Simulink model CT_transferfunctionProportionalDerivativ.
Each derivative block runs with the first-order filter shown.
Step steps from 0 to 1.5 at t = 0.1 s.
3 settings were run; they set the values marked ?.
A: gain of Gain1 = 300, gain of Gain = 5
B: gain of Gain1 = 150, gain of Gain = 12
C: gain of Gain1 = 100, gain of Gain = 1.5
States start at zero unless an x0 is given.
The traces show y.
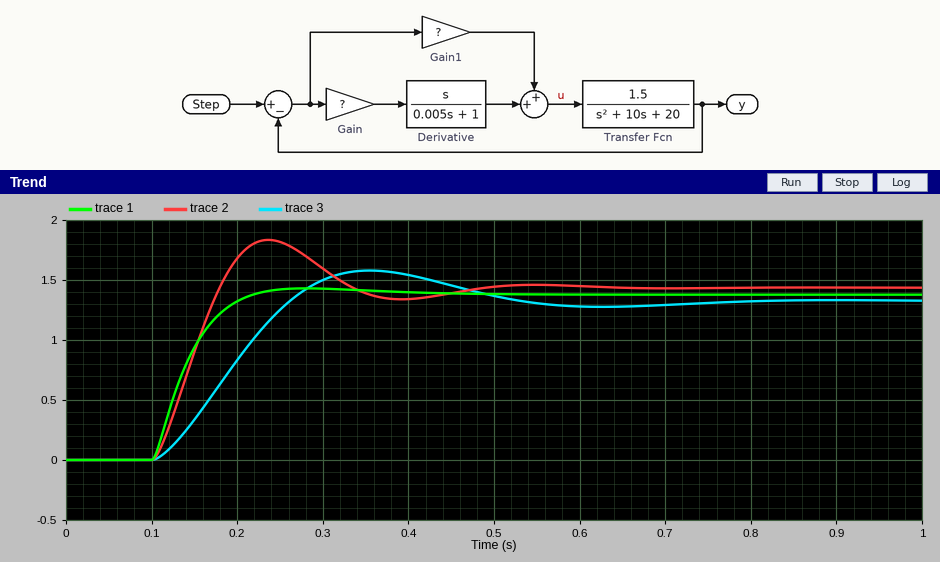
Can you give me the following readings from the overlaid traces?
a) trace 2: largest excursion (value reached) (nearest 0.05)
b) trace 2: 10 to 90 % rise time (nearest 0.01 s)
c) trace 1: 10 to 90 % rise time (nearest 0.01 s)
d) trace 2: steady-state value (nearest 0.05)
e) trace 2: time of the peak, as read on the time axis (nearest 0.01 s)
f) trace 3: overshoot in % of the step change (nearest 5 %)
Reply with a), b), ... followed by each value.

a) 1.85
b) 0.06 s
c) 0.07 s
d) 1.45
e) 0.24 s
f) 20 %
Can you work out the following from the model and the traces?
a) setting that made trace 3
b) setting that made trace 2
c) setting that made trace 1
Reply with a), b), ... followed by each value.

a) C
b) A
c) B
